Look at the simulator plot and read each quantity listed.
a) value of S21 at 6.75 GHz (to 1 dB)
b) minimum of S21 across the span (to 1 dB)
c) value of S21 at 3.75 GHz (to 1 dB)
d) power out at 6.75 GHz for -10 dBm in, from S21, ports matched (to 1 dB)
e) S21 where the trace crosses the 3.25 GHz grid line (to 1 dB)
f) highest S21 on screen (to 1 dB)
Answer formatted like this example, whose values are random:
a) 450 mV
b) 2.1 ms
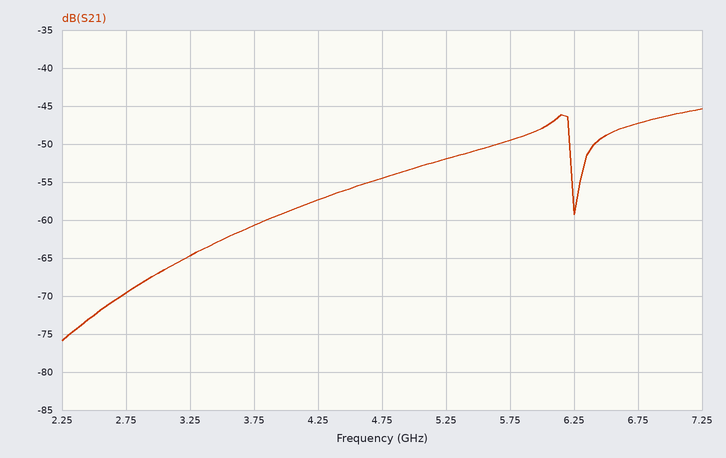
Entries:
a) -47 dB
b) -76 dB
c) -61 dB
d) -57 dBm
e) -65 dB
f) -45 dB
